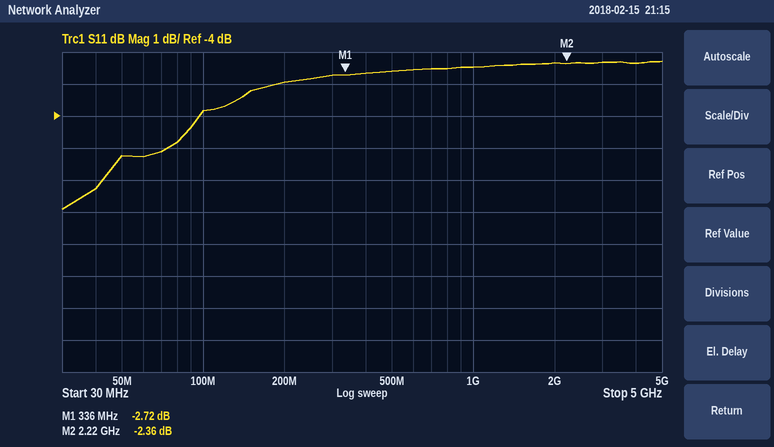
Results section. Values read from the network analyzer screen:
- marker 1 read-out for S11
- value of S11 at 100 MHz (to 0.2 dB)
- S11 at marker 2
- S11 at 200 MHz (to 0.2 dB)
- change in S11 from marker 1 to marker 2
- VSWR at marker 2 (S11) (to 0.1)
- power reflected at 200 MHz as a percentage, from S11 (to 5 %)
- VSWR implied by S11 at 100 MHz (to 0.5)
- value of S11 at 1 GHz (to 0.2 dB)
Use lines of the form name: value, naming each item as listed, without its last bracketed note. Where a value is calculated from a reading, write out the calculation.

marker 1 read-out for S11: -2.72 dB
value of S11 at 100 MHz: -3.8 dB
S11 at marker 2: -2.36 dB
S11 at 200 MHz: -3.0 dB
change in S11 from marker 1 to marker 2: -2.36 − (-2.72) = 0.36 dB
VSWR at marker 2 (S11): (1 + 0.7621)/(1 − 0.7621) ≈ 7.4
power reflected at 200 MHz as a percentage, from S11: 10^(-3/10) ≈ 50 %
VSWR implied by S11 at 100 MHz: |Γ| = 10^(-3.8/20) = 0.6457; VSWR = (1 + 0.6457)/(1 − 0.6457) ≈ 4.64, so 4.5 to the nearest 0.5
value of S11 at 1 GHz: -2.4 dB
